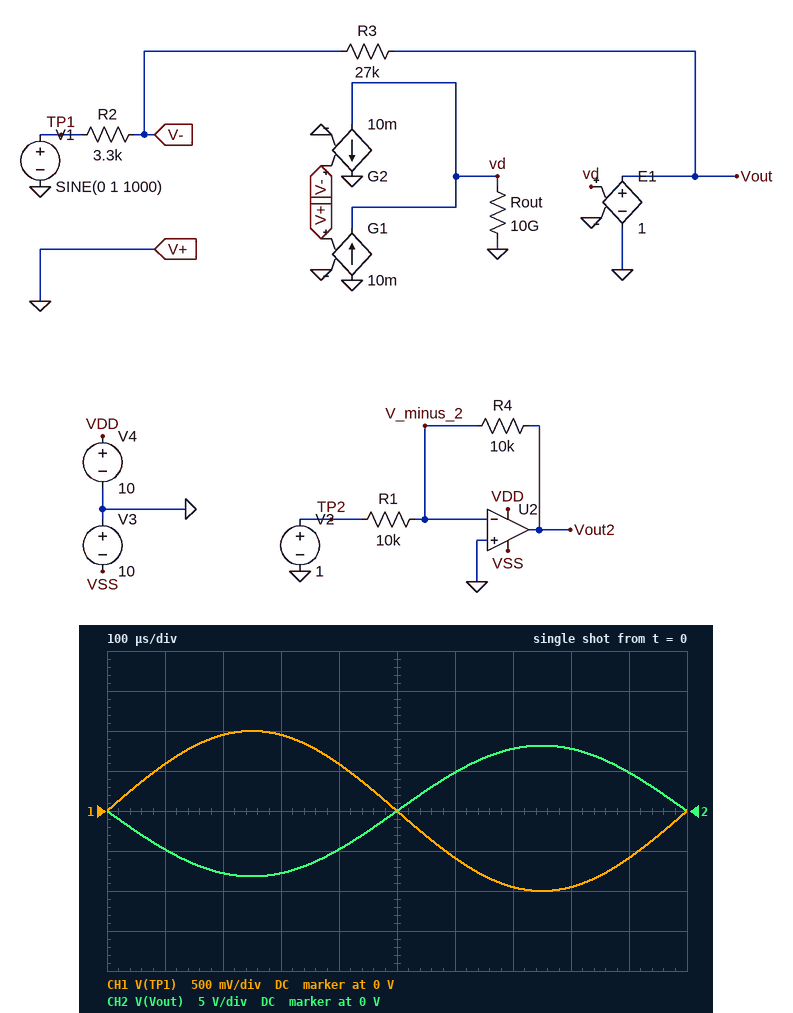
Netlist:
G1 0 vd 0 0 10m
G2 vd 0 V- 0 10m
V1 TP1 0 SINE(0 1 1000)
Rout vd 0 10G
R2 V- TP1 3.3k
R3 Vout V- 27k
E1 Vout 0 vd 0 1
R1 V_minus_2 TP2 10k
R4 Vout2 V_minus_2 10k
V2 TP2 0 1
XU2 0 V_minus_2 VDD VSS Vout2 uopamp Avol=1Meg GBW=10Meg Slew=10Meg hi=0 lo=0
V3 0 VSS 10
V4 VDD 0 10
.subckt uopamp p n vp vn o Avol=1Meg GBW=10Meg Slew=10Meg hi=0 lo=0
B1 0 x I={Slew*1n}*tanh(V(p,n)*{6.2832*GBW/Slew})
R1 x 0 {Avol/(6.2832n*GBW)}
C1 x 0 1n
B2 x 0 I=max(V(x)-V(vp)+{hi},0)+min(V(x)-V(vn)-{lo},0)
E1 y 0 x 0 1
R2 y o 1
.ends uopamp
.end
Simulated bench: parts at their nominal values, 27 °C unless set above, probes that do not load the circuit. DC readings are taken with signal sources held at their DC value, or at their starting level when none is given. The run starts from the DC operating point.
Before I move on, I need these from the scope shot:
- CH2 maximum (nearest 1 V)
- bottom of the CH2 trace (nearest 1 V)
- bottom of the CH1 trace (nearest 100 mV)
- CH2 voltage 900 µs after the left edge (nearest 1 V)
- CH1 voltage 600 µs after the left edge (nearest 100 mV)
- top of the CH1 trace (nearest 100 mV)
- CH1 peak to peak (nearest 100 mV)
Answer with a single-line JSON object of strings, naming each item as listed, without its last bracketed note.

{"CH2 maximum": "8 V", "bottom of the CH2 trace": "-8 V", "bottom of the CH1 trace": "-1.0 V", "CH2 voltage 900 µs after the left edge": "5 V", "CH1 voltage 600 µs after the left edge": "-600 mV", "top of the CH1 trace": "1.0 V", "CH1 peak to peak": "2.0 V"}
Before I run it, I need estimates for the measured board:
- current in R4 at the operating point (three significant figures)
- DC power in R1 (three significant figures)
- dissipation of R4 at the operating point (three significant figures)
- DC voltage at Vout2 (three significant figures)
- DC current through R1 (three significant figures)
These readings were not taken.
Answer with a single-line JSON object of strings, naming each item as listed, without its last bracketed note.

{"current in R4 at the operating point": "100 µA", "DC power in R1": "100 µW", "dissipation of R4 at the operating point": "100 µW", "DC voltage at Vout2": "-1.00 V", "DC current through R1": "100 µA"}
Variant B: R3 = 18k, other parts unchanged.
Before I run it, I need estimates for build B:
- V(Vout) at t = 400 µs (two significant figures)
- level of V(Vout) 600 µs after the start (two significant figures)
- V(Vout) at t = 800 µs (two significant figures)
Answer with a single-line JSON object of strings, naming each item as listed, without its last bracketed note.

{"V(Vout) at t = 400 µs": "-3.2 V", "level of V(Vout) 600 µs after the start": "3.2 V", "V(Vout) at t = 800 µs": "5.2 V"}
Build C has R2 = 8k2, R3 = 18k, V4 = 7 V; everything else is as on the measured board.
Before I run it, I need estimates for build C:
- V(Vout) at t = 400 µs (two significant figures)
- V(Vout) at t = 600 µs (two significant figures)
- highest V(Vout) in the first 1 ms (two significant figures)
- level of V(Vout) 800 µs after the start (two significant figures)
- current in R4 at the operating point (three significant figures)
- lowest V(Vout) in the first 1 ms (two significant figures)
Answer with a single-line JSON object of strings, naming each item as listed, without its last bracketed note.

{"V(Vout) at t = 400 µs": "-1.3 V", "V(Vout) at t = 600 µs": "1.3 V", "highest V(Vout) in the first 1 ms": "2.2 V", "level of V(Vout) 800 µs after the start": "2.1 V", "current in R4 at the operating point": "100 µA", "lowest V(Vout) in the first 1 ms": "-2.2 V"}
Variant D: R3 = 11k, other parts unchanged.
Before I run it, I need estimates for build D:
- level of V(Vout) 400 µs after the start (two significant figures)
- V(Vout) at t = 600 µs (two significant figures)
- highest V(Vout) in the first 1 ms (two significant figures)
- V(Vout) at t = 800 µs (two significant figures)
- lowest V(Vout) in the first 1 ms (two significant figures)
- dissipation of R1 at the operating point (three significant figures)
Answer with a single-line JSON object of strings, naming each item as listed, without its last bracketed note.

{"level of V(Vout) 400 µs after the start": "-2.0 V", "V(Vout) at t = 600 µs": "2.0 V", "highest V(Vout) in the first 1 ms": "3.3 V", "V(Vout) at t = 800 µs": "3.2 V", "lowest V(Vout) in the first 1 ms": "-3.3 V", "dissipation of R1 at the operating point": "100 µW"}
